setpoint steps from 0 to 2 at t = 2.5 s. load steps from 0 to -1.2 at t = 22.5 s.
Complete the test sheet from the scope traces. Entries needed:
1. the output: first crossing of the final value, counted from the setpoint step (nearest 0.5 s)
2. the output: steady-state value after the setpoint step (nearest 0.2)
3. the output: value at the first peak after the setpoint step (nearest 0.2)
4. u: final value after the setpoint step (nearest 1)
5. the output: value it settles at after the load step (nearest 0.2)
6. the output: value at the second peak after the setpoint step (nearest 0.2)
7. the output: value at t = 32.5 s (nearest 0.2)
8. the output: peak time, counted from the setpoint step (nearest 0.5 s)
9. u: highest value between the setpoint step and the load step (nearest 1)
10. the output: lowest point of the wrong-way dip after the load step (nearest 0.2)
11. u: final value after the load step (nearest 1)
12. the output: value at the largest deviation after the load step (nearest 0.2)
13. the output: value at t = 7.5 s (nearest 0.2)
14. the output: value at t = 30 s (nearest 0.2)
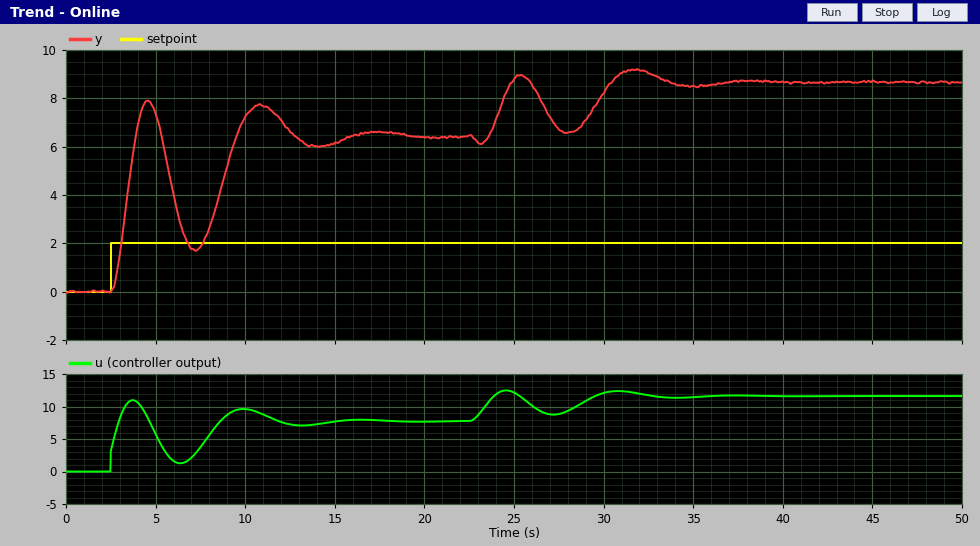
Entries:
1.5 s
6.4
7.8
8
8.6
7.8
9.0
2.0 s
11
6.2
12
9.2
1.8
8.2
